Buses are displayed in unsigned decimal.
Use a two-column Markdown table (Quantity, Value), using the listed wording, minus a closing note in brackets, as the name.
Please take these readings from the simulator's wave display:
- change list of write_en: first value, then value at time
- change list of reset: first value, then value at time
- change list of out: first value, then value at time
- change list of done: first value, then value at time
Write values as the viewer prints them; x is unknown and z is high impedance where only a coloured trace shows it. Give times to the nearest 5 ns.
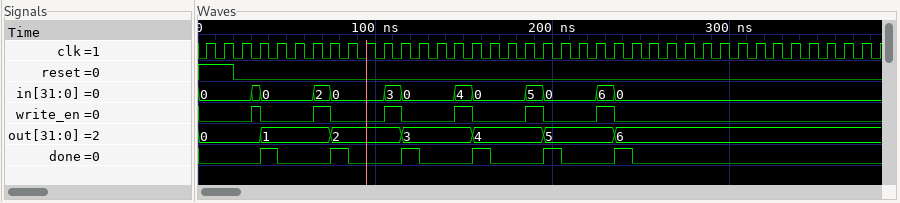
| Quantity | Value |
|---|---|
| change list of write_en: first value, then value at time | 0, 1 at 30 ns, 0 at 35 ns, 1 at 65 ns, 0 at 75 ns, 1 at 105 ns, 0 at 115 ns, 1 at 145 ns, 0 at 155 ns, 1 at 185 ns, 0 at 195 ns, 1 at 225 ns, 0 at 235 ns |
| change list of reset: first value, then value at time | 1, 0 at 20 ns |
| change list of out: first value, then value at time | 0, 1 at 35 ns, 2 at 75 ns, 3 at 115 ns, 4 at 155 ns, 5 at 195 ns, 6 at 235 ns |
| change list of done: first value, then value at time | 0, 1 at 35 ns, 0 at 45 ns, 1 at 75 ns, 0 at 85 ns, 1 at 115 ns, 0 at 125 ns, 1 at 155 ns, 0 at 165 ns, 1 at 195 ns, 0 at 205 ns, 1 at 235 ns, 0 at 245 ns |
